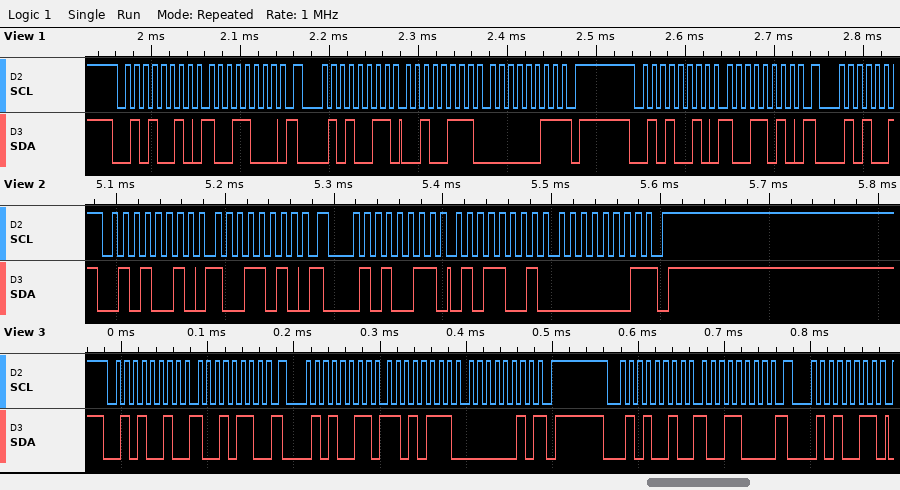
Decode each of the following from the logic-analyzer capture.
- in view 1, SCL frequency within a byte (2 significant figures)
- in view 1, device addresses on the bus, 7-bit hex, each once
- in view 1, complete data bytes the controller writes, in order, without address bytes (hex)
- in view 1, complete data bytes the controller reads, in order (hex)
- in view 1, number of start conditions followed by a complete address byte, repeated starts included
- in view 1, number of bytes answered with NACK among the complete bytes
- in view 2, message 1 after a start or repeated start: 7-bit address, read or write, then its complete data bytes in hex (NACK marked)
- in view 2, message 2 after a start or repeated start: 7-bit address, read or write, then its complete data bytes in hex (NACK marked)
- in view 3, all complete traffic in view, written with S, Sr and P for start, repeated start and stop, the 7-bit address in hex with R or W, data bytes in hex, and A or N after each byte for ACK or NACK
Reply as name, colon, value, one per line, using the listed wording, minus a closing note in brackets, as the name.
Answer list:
in view 1, SCL frequency within a byte: 100 kHz
in view 1, device addresses on the bus, 7-bit hex, each once: 0x29
in view 1, complete data bytes the controller writes, in order, without address bytes: 98 9A
in view 1, complete data bytes the controller reads, in order: 27 03
in view 1, number of start conditions followed by a complete address byte, repeated starts included: 3
in view 1, number of bytes answered with NACK among the complete bytes: 1
in view 2, message 1 after a start or repeated start: 7-bit address, read or write, then its complete data bytes in hex: 0x29 write: 9A
in view 2, message 2 after a start or repeated start: 7-bit address, read or write, then its complete data bytes in hex: 0x29 read: 59 01 NACK
in view 3, all complete traffic in view, written with S, Sr and P for start, repeated start and stop, the 7-bit address in hex with R or W, data bytes in hex, and A or N after each byte for ACK or NACK: S 29W A 96 A Sr 29R A D7 A 02 N P S 29W A 98 A Sr 29R A
